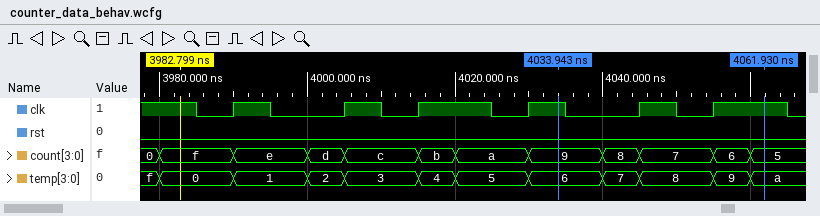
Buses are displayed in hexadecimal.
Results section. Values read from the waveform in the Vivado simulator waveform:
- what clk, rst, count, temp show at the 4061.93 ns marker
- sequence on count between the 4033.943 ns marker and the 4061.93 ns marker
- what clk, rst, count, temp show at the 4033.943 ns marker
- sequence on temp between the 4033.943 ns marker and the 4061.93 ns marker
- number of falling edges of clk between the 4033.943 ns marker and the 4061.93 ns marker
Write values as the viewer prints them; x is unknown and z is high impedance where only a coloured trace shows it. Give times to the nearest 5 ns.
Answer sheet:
clk=1, rst=0, count=5, temp=a
9, 8, 7, 6, 5
clk=1, rst=0, count=9, temp=6
6, 7, 8, 9, a
2
